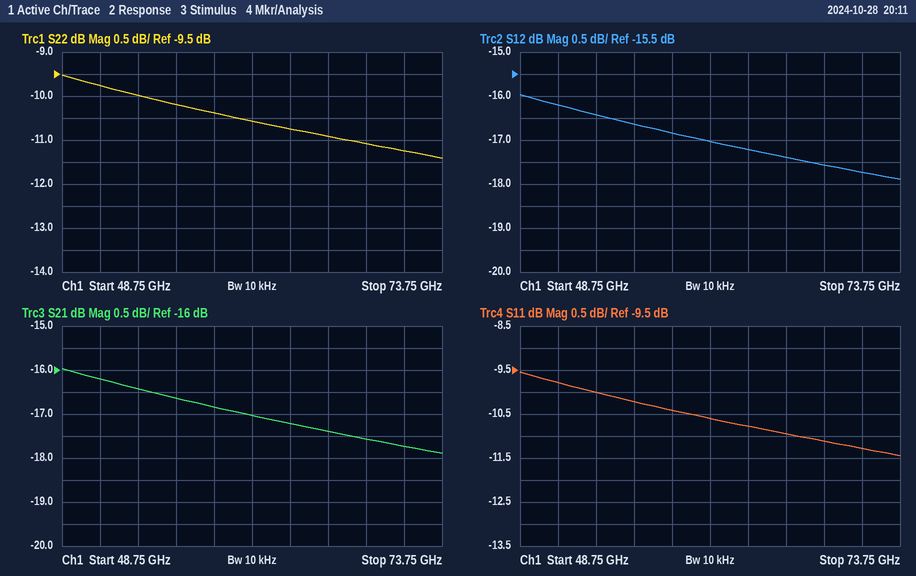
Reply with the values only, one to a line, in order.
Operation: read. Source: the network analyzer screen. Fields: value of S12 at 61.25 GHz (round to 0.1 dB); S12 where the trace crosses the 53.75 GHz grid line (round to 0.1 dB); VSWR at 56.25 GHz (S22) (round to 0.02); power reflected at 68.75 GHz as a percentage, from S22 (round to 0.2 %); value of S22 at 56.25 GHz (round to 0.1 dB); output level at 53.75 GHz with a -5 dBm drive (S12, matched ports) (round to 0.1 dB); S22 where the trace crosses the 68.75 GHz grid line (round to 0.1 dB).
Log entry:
-17.0 dB
-16.4 dB
1.90
7.8 %
-10.2 dB
-21.4 dBm
-11.1 dB
